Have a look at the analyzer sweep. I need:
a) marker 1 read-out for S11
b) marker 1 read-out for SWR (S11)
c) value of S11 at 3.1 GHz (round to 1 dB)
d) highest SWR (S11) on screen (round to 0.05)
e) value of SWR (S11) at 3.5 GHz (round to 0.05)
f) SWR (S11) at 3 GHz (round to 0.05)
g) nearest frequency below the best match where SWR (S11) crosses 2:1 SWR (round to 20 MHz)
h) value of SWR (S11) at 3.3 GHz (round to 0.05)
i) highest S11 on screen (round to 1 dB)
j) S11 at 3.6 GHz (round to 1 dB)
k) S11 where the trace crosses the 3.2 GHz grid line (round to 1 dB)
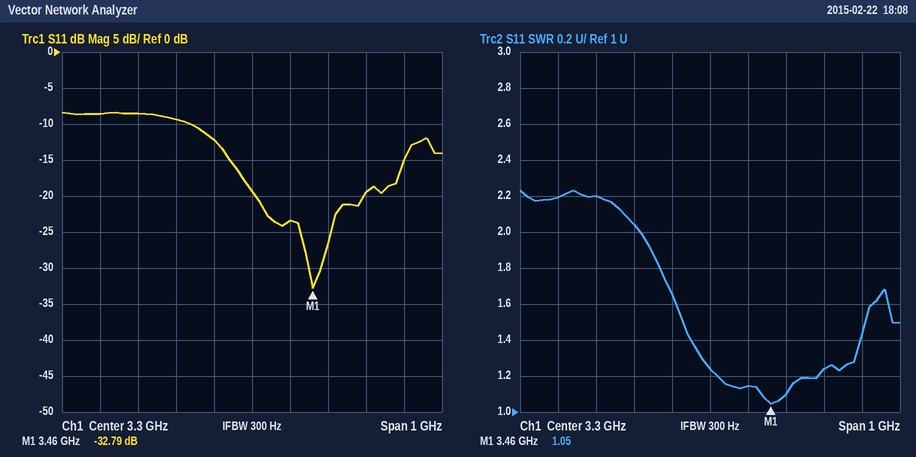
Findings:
-32.79 dB
1.05
-9 dB
2.25
1.10
2.20
3.12 GHz
1.25
-8 dB
-19 dB
-12 dB
